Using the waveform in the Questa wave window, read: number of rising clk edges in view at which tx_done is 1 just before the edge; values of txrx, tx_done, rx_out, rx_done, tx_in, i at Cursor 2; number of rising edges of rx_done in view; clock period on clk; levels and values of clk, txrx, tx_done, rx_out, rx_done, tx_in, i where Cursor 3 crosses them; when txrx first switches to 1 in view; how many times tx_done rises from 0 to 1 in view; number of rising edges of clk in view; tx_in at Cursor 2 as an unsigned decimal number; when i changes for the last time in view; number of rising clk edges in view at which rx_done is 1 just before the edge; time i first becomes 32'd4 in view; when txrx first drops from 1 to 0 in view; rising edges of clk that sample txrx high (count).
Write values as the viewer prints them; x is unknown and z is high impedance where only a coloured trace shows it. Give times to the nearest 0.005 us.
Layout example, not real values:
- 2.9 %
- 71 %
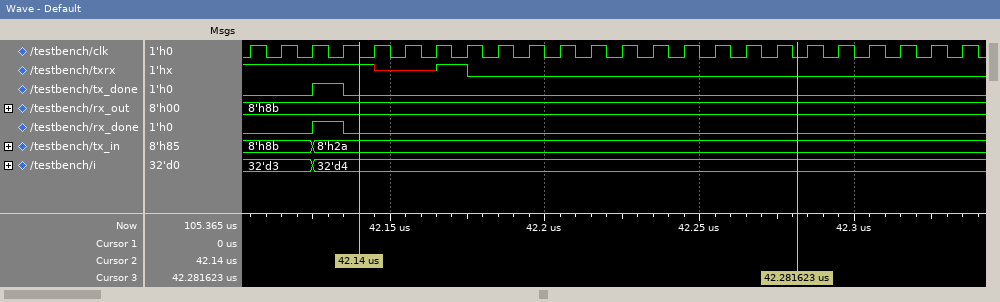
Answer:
- 1
- txrx=1, tx_done=0, rx_out=8'h8b, rx_done=0, tx_in=8'h2a, i=32'd4
- 1
- 0.01 us
- clk=0, txrx=0, tx_done=0, rx_out=8'h8b, rx_done=0, tx_in=8'h2a, i=32'd4
- 42.165 us
- 1
- 24
- 42
- 42.125 us
- 1
- 42.125 us
- 42.175 us
- 6
